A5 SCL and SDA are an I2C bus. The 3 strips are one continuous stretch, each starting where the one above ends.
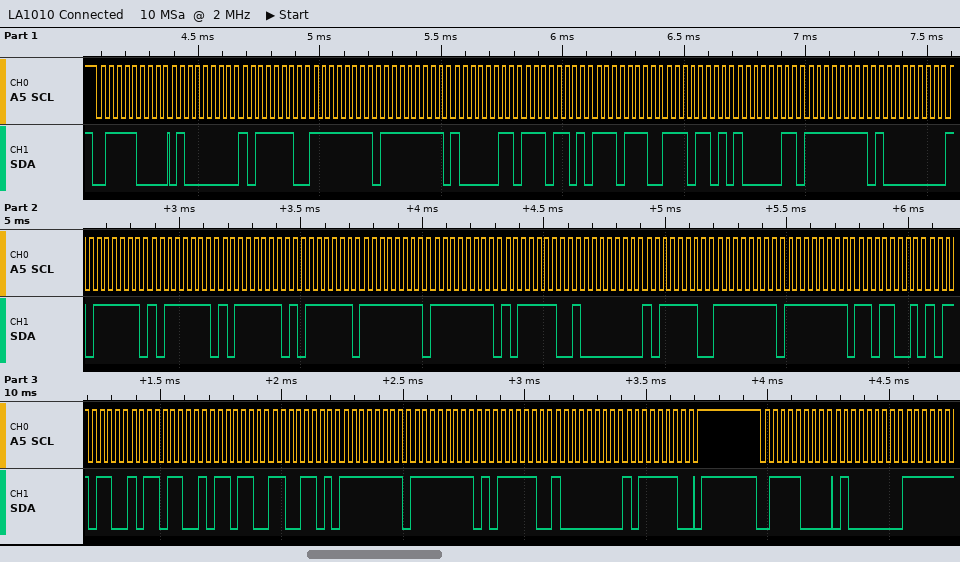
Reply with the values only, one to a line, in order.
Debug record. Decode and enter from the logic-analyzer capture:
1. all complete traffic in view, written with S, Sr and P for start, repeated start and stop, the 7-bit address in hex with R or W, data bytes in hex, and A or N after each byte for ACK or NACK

S 3CW A 40 A BE A FF A FF A 83 A ED A EE A ED A 83 A FF A 80 A BF A BF A BF A BF A FF A FF A BE A 80 A BE A FF A FF A D9 A B6 A B6 A B6 A CD A FF A FF A BE A 80 A BE A P S 3CW A 40 A
